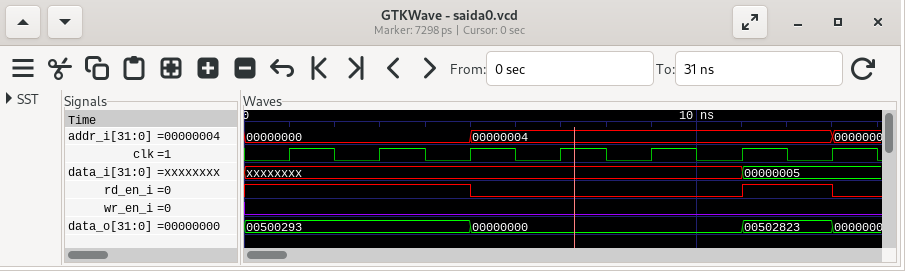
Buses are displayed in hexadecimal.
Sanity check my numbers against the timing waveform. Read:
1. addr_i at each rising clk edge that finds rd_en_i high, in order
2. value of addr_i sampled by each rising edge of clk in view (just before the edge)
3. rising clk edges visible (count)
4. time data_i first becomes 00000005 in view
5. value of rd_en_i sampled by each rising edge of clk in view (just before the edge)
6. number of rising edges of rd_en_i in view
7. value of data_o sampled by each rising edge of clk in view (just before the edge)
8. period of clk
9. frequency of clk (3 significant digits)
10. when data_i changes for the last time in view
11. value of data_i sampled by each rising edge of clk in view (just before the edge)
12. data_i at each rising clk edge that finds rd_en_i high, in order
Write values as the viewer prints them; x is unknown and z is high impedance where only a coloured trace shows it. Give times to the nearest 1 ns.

00000000, 00000000, 00000000, 00000004
00000000, 00000000, 00000000, 00000004, 00000004, 00000004, 00000004
7
11 ns
1 1 1 0 0 0 1
1
00500293, 00500293, 00500293, 00000000, 00000000, 00000000, 00502823
2 ns
500 MHz
11 ns
xxxxxxxx, xxxxxxxx, xxxxxxxx, xxxxxxxx, xxxxxxxx, xxxxxxxx, 00000005
xxxxxxxx, xxxxxxxx, xxxxxxxx, 00000005
